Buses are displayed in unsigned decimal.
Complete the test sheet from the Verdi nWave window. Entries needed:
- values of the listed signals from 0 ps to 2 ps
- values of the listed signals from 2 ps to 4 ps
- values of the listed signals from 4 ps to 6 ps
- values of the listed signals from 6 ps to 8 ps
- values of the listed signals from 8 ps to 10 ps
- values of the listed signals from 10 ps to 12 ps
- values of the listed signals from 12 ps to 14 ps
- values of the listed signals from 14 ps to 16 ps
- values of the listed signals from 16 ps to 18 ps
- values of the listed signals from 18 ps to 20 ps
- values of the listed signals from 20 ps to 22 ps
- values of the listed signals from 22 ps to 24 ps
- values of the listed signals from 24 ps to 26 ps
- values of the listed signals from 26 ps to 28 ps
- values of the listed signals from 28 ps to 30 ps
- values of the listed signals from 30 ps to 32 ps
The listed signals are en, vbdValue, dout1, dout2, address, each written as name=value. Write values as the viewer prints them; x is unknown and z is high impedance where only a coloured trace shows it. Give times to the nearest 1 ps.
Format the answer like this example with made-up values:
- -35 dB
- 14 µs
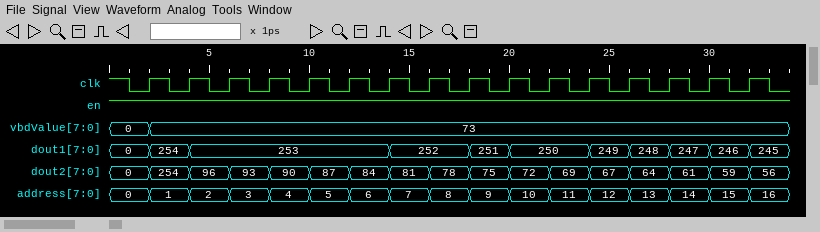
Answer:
- en=1, vbdValue=0, dout1=0, dout2=0, address=0
- en=1, vbdValue=73, dout1=254, dout2=254, address=1
- en=1, vbdValue=73, dout1=253, dout2=96, address=2
- en=1, vbdValue=73, dout1=253, dout2=93, address=3
- en=1, vbdValue=73, dout1=253, dout2=90, address=4
- en=1, vbdValue=73, dout1=253, dout2=87, address=5
- en=1, vbdValue=73, dout1=253, dout2=84, address=6
- en=1, vbdValue=73, dout1=252, dout2=81, address=7
- en=1, vbdValue=73, dout1=252, dout2=78, address=8
- en=1, vbdValue=73, dout1=251, dout2=75, address=9
- en=1, vbdValue=73, dout1=250, dout2=72, address=10
- en=1, vbdValue=73, dout1=250, dout2=69, address=11
- en=1, vbdValue=73, dout1=249, dout2=67, address=12
- en=1, vbdValue=73, dout1=248, dout2=64, address=13
- en=1, vbdValue=73, dout1=247, dout2=61, address=14
- en=1, vbdValue=73, dout1=246, dout2=59, address=15
